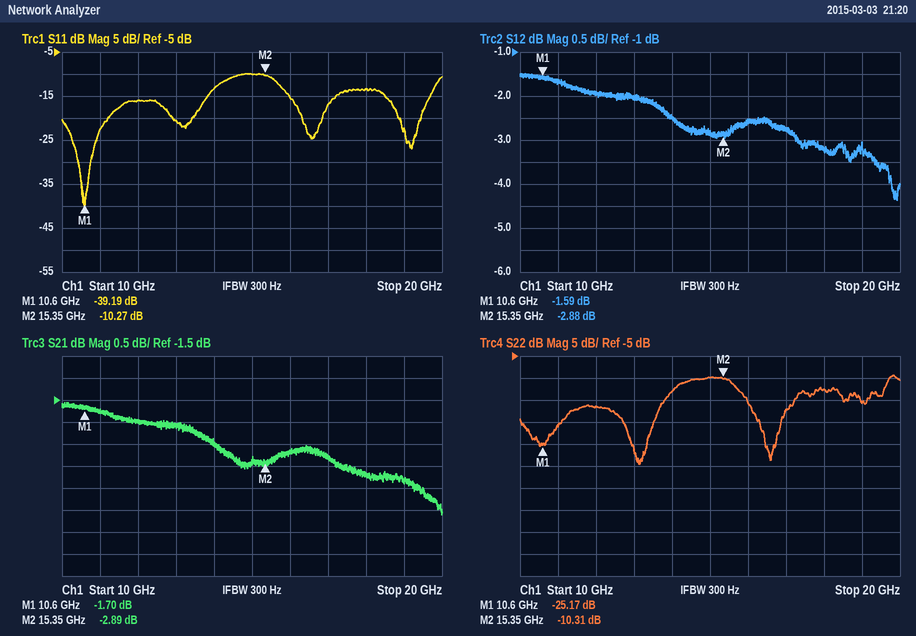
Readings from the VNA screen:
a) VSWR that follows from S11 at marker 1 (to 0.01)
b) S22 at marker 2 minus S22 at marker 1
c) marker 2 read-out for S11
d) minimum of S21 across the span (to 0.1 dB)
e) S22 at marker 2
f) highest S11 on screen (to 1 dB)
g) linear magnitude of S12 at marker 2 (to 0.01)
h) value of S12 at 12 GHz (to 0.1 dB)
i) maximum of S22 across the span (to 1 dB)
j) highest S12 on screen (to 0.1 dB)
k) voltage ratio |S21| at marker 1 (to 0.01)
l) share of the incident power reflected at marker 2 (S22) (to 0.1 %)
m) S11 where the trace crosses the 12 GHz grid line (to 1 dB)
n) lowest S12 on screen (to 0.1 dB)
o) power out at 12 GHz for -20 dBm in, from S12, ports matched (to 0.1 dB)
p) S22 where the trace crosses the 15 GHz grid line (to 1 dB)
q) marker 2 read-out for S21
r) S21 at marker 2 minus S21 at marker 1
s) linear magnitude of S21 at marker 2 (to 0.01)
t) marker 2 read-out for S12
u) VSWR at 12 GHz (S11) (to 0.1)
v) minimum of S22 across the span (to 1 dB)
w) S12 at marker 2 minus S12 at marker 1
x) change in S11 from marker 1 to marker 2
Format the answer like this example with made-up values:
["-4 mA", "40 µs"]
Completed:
["1.02", "14.86 dB", "-10.27 dB", "-4.1 dB", "-10.31 dB", "-10 dB", "0.72", "-1.9 dB", "-9 dB", "-1.5 dB", "0.82", "9.3 %", "-16 dB", "-4.4 dB", "-21.9 dBm", "-10 dB", "-2.89 dB", "-1.19 dB", "0.72", "-2.88 dB", "1.4", "-30 dB", "-1.29 dB", "28.92 dB"]
